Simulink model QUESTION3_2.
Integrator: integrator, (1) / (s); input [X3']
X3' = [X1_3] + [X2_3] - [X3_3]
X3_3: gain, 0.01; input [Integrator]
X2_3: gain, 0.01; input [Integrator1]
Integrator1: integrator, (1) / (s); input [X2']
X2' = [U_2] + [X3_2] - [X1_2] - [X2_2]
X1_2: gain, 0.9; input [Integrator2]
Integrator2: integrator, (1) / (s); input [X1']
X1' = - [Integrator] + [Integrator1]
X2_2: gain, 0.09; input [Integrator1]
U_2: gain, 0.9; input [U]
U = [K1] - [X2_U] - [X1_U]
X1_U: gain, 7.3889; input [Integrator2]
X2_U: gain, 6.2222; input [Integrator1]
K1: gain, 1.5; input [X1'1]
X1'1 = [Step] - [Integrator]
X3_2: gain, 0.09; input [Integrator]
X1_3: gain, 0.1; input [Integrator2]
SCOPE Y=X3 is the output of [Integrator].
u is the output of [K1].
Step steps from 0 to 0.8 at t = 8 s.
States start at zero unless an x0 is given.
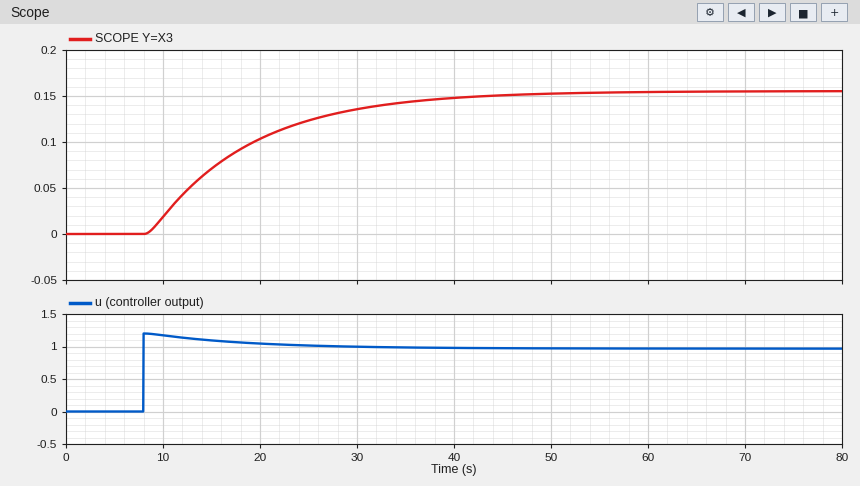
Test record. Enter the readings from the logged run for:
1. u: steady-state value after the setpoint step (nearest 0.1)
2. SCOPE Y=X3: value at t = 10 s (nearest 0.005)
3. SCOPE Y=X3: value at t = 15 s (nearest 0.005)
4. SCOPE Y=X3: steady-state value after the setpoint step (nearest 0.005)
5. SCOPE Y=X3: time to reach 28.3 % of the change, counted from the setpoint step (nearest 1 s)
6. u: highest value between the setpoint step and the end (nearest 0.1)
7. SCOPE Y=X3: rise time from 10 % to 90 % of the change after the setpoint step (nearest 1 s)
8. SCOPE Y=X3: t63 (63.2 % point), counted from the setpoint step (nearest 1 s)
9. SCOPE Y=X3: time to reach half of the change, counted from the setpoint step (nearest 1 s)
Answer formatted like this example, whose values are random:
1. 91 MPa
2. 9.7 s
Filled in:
1. 1.0
2. 0.020
3. 0.070
4. 0.155
5. 4 s
6. 1.2
7. 23 s
8. 11 s
9. 8 s
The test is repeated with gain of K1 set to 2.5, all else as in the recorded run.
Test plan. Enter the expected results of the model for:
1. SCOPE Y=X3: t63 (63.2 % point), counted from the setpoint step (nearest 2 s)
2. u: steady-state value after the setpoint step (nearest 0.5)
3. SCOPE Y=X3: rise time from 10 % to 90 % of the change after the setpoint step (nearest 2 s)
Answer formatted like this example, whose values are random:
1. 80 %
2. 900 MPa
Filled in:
1. 10 s
2. 1.5
3. 20 s
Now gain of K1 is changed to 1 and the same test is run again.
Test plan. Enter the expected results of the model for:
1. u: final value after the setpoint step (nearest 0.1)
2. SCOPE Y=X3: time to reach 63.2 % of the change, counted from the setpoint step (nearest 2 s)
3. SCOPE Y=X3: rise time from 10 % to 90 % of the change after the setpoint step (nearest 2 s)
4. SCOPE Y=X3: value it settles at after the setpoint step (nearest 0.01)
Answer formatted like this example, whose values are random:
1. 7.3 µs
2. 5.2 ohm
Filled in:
1. 0.7
2. 12 s
3. 24 s
4. 0.11
